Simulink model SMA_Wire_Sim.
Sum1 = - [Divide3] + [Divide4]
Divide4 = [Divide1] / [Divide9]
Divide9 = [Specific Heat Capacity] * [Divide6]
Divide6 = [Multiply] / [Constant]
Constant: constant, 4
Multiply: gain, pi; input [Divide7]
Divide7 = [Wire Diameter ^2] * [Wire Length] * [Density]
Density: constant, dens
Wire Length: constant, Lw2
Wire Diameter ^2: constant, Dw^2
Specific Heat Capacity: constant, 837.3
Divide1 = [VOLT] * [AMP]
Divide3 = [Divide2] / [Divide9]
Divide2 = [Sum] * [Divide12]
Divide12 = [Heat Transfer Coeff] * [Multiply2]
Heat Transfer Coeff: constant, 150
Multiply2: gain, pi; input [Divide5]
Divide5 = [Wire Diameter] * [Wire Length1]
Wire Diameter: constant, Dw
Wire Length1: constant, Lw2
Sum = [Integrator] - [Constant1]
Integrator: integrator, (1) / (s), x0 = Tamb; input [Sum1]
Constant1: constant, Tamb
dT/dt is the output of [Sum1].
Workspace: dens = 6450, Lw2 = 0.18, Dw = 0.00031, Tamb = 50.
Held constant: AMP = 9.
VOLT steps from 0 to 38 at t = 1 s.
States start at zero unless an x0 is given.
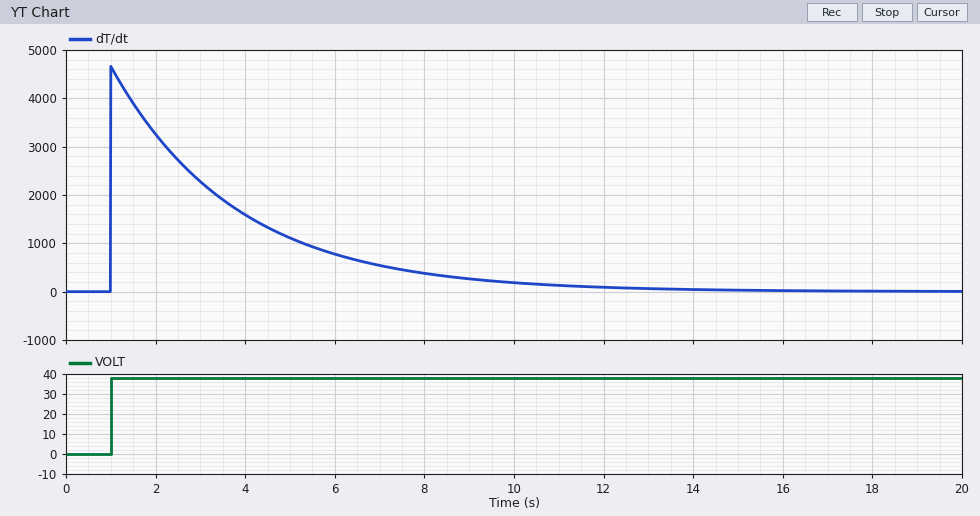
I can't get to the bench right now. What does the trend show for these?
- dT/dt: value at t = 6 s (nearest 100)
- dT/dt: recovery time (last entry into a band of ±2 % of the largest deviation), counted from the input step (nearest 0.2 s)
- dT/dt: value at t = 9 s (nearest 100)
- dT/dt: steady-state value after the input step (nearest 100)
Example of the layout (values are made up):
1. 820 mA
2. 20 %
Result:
1. 800
2. 11.0 s
3. 300
4. 0
